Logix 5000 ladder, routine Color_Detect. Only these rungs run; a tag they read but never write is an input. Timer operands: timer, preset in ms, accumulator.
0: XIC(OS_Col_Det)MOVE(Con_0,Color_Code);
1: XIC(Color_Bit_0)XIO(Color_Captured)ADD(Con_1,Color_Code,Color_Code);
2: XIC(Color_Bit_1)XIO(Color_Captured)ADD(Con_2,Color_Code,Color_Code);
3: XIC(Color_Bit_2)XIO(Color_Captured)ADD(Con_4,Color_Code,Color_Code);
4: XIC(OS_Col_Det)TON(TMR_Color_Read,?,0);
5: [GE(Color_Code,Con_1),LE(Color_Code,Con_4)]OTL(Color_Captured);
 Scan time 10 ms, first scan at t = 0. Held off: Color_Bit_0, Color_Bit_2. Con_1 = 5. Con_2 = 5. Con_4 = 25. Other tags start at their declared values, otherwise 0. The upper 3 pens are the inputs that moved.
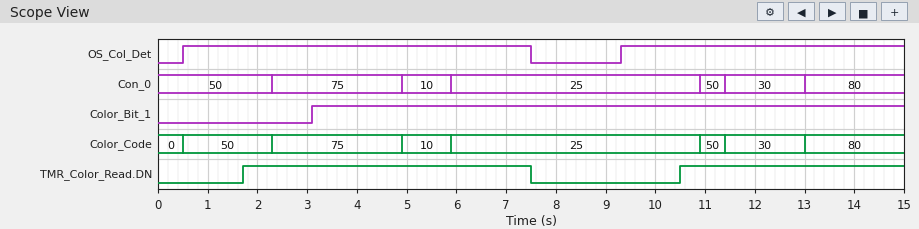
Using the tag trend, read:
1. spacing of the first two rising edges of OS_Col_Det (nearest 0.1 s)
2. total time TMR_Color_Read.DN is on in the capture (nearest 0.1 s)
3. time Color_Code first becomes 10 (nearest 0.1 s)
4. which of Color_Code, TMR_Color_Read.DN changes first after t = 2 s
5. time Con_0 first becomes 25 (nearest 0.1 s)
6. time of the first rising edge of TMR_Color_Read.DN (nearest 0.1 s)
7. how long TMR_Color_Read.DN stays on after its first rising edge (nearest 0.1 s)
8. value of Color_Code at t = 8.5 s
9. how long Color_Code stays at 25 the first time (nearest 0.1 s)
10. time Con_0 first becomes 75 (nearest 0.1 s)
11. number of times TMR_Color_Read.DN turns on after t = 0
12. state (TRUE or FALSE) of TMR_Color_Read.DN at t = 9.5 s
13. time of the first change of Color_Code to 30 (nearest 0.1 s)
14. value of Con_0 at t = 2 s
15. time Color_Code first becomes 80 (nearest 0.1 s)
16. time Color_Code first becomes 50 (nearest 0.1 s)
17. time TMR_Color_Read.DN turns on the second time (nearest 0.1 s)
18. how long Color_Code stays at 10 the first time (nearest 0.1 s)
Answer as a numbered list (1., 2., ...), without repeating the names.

1. 8.8 s
2. 10.3 s
3. 4.9 s
4. Color_Code
5. 5.9 s
6. 1.7 s
7. 5.8 s
8. 25
9. 5.0 s
10. 2.3 s
11. 2
12. FALSE
13. 11.4 s
14. 50
15. 13.0 s
16. 0.5 s
17. 10.5 s
18. 1.0 s
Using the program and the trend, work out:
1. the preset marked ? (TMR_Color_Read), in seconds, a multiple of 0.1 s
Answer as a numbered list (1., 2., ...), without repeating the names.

1. 1.2 s
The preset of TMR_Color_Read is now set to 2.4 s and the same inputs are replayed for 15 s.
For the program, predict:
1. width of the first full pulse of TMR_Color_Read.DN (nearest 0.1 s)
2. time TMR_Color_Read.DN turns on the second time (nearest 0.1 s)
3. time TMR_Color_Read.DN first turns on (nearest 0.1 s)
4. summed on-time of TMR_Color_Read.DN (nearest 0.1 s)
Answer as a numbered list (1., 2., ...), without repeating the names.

1. 4.6 s
2. 11.7 s
3. 2.9 s
4. 7.9 s
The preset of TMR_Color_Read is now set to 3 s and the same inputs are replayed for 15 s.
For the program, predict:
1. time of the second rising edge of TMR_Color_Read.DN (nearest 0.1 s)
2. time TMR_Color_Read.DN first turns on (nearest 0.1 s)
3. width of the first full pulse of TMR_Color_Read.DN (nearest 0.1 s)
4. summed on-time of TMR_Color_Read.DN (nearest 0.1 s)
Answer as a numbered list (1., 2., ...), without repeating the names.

1. 12.3 s
2. 3.5 s
3. 4.0 s
4. 6.7 s
